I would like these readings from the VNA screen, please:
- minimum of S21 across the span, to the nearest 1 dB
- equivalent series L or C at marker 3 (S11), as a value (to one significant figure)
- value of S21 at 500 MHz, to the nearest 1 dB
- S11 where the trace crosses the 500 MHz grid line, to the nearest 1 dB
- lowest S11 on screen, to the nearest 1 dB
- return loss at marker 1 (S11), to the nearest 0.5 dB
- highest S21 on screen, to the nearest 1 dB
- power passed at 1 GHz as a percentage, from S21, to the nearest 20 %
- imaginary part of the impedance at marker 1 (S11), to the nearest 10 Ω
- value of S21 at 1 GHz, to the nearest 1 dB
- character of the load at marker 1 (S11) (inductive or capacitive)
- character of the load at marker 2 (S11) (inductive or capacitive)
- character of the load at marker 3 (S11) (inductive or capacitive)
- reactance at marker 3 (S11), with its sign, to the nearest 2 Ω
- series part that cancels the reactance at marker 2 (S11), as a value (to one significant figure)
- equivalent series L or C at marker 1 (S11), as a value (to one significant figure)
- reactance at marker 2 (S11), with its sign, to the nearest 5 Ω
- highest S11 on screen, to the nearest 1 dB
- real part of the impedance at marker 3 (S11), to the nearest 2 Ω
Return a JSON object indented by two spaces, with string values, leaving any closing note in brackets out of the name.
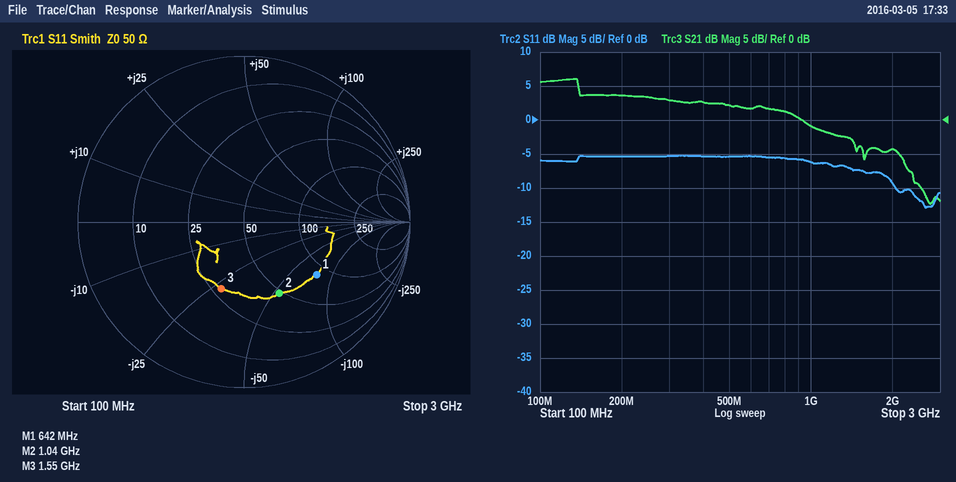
{
  "minimum of S21 across the span, to the nearest 1 dB": "-12 dB",
  "equivalent series L or C at marker 3 (S11), as a value": "4 pF",
  "value of S21 at 500 MHz, to the nearest 1 dB": "2 dB",
  "S11 where the trace crosses the 500 MHz grid line, to the nearest 1 dB": "-5 dB",
  "lowest S11 on screen, to the nearest 1 dB": "-13 dB",
  "return loss at marker 1 (S11), to the nearest 0.5 dB": "5.5 dB",
  "highest S21 on screen, to the nearest 1 dB": "6 dB",
  "power passed at 1 GHz as a percentage, from S21, to the nearest 20 %": "80 %",
  "imaginary part of the impedance at marker 1 (S11), to the nearest 10 Ω": "-80 Ω",
  "value of S21 at 1 GHz, to the nearest 1 dB": "-1 dB",
  "character of the load at marker 1 (S11)": "capacitive",
  "character of the load at marker 2 (S11)": "capacitive",
  "character of the load at marker 3 (S11)": "capacitive",
  "reactance at marker 3 (S11), with its sign, to the nearest 2 Ω": "-28 Ω",
  "series part that cancels the reactance at marker 2 (S11), as a value": "8 nH",
  "equivalent series L or C at marker 1 (S11), as a value": "3 pF",
  "reactance at marker 2 (S11), with its sign, to the nearest 5 Ω": "-55 Ω",
  "highest S11 on screen, to the nearest 1 dB": "-5 dB",
  "real part of the impedance at marker 3 (S11), to the nearest 2 Ω": "28 Ω"
}
